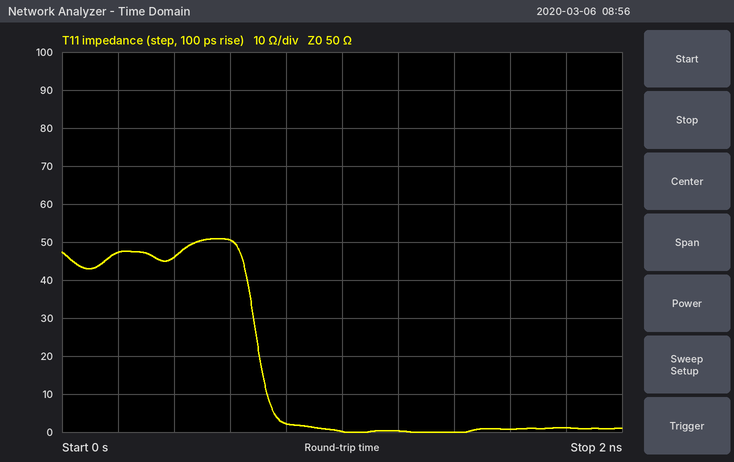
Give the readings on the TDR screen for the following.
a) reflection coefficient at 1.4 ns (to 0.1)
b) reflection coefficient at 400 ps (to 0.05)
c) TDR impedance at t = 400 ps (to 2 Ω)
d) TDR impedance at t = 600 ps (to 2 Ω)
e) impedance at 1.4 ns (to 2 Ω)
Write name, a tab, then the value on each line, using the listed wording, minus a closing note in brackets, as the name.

reflection coefficient at 1.4 ns	-1.0
reflection coefficient at 400 ps	-0.05
TDR impedance at t = 400 ps	46 Ω
TDR impedance at t = 600 ps	50 Ω
impedance at 1.4 ns	0 Ω
